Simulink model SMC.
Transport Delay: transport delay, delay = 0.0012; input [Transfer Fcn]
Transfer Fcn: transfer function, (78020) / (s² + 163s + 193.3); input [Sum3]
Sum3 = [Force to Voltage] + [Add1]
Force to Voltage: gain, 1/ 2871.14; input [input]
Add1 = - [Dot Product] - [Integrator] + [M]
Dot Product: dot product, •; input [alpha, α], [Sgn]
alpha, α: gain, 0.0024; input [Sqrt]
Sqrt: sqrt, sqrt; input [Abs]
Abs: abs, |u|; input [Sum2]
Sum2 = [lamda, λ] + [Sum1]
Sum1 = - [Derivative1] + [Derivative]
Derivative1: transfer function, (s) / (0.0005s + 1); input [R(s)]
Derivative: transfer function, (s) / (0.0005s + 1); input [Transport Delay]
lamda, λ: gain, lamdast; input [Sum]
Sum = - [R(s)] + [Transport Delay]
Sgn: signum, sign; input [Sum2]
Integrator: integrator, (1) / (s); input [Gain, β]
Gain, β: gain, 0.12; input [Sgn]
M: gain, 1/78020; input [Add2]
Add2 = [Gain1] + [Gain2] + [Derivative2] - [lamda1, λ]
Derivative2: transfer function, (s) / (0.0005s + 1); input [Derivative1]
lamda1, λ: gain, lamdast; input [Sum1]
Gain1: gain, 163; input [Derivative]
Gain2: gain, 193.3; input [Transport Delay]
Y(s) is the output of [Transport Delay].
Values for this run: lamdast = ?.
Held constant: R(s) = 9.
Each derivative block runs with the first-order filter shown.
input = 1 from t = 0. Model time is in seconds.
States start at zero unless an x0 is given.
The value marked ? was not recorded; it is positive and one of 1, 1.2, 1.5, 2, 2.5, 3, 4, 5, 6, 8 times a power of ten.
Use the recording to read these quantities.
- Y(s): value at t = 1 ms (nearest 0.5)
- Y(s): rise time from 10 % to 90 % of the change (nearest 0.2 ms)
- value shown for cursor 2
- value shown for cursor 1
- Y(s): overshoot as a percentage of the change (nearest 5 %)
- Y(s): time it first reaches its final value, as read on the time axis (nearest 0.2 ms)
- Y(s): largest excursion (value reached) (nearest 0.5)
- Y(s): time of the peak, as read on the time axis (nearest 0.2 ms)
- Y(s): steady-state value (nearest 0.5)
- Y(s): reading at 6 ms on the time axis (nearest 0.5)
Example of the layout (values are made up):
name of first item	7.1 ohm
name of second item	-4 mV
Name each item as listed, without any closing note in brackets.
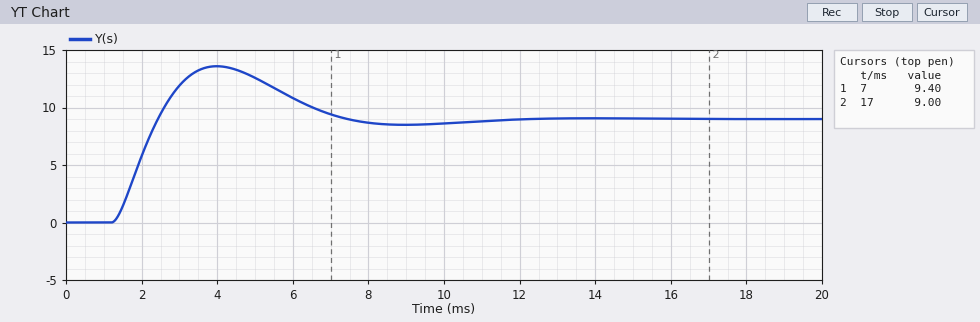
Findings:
Y(s): value at t = 1 ms	0.0
Y(s): rise time from 10 % to 90 % of the change	0.8 ms
value shown for cursor 2	9.00
value shown for cursor 1	9.40
Y(s): overshoot as a percentage of the change	50 %
Y(s): time it first reaches its final value, as read on the time axis	2.4 ms
Y(s): largest excursion (value reached)	13.5
Y(s): time of the peak, as read on the time axis	4.0 ms
Y(s): steady-state value	9.0
Y(s): reading at 6 ms on the time axis	11.0
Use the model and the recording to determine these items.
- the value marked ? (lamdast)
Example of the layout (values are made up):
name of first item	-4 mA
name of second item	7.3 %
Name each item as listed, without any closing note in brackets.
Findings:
the value marked ?	500
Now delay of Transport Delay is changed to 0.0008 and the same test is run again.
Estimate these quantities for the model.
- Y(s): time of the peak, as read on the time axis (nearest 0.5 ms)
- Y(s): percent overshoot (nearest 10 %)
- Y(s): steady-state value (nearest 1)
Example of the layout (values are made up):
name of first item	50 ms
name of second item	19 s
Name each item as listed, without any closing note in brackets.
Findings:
Y(s): time of the peak, as read on the time axis	3.5 ms
Y(s): percent overshoot	40 %
Y(s): steady-state value	9
